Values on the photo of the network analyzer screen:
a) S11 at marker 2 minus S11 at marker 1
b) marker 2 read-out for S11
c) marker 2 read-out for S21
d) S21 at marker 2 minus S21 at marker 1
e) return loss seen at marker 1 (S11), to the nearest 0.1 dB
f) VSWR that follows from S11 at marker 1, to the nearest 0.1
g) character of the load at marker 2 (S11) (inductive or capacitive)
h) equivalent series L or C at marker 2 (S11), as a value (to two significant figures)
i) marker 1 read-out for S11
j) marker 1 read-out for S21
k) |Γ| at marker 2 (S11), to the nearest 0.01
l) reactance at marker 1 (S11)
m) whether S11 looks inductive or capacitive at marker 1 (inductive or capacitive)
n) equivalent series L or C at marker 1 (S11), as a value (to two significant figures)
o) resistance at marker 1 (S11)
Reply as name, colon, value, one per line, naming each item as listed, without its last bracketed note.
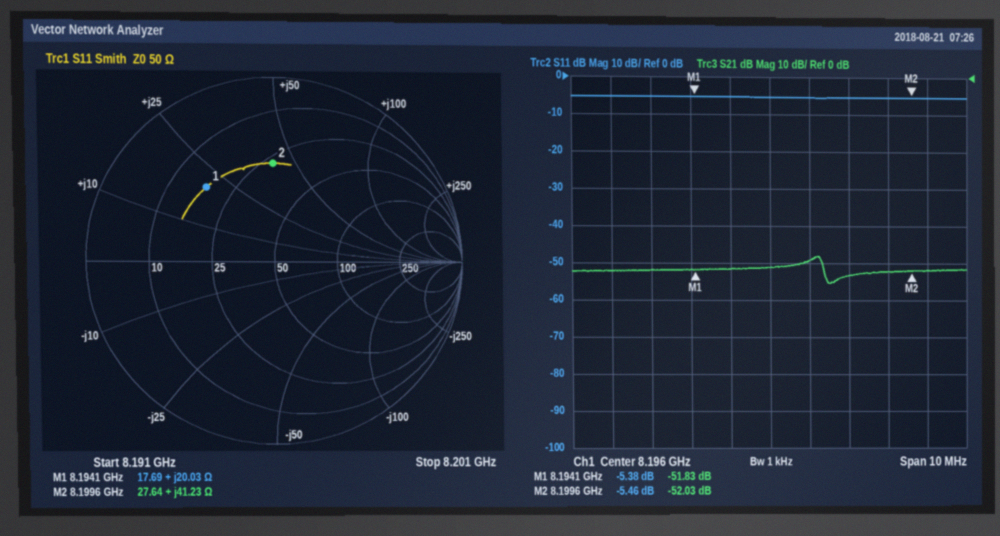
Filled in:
S11 at marker 2 minus S11 at marker 1: -0.08 dB
marker 2 read-out for S11: -5.46 dB
marker 2 read-out for S21: -52.03 dB
S21 at marker 2 minus S21 at marker 1: -0.20 dB
return loss seen at marker 1 (S11), to the nearest 0.1 dB: 5.4 dB
VSWR that follows from S11 at marker 1, to the nearest 0.1: 3.3
character of the load at marker 2 (S11): inductive
equivalent series L or C at marker 2 (S11), as a value: 800 pH
marker 1 read-out for S11: -5.38 dB
marker 1 read-out for S21: -51.83 dB
|Γ| at marker 2 (S11), to the nearest 0.01: 0.53
reactance at marker 1: +20.03 Ω
whether S11 looks inductive or capacitive at marker 1: inductive
equivalent series L or C at marker 1 (S11), as a value: 390 pH
resistance at marker 1: 17.69 Ω
